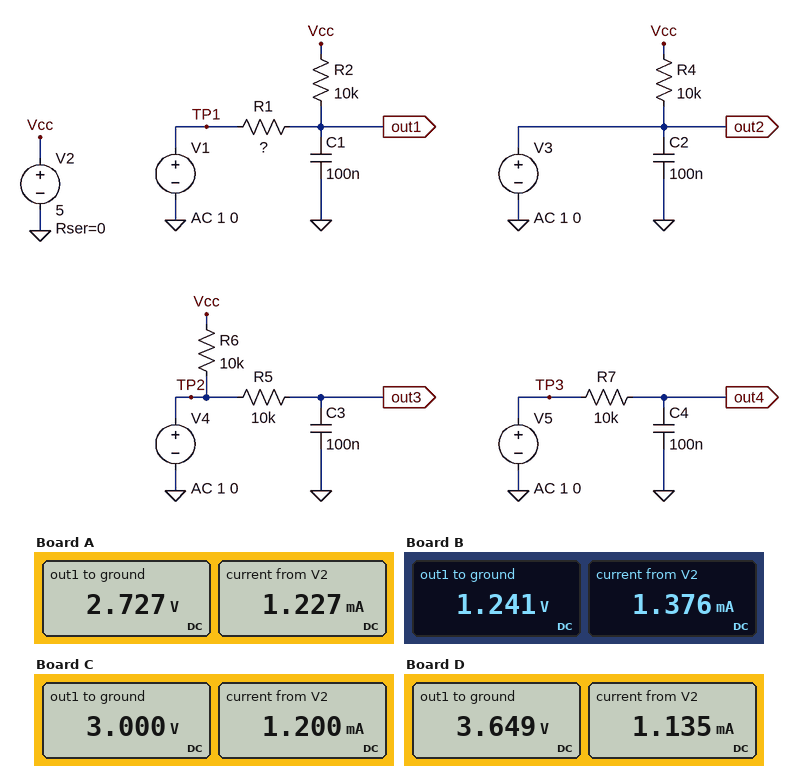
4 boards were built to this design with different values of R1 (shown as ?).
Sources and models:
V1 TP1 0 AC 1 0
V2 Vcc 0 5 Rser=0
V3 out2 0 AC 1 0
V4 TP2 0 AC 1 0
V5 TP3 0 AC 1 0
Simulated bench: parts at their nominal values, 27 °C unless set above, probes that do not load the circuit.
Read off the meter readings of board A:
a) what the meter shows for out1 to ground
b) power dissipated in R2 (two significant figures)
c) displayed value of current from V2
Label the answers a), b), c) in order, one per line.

a) 2.727 V
b) 520 µW
c) 1.227 mA
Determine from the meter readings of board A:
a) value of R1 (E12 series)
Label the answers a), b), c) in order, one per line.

a) 12 kΩ
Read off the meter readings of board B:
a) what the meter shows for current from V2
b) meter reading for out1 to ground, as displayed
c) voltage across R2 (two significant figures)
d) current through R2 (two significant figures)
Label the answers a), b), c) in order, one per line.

a) 1.376 mA
b) 1.241 V
c) 3.8 V
d) 380 µA
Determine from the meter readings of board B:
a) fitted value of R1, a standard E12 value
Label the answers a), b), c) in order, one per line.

a) 3.3 kΩ
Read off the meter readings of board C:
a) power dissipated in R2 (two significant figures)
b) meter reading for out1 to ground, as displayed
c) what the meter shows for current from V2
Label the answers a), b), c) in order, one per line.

a) 400 µW
b) 3.000 V
c) 1.200 mA
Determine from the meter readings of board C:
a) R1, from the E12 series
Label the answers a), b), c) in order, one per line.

a) 15 kΩ
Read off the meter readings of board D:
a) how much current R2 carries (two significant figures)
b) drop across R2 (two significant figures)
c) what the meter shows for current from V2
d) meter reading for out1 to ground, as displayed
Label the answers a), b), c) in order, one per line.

a) 140 µA
b) 1.4 V
c) 1.135 mA
d) 3.649 V
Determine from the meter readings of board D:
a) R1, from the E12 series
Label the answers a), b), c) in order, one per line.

a) 27 kΩ
